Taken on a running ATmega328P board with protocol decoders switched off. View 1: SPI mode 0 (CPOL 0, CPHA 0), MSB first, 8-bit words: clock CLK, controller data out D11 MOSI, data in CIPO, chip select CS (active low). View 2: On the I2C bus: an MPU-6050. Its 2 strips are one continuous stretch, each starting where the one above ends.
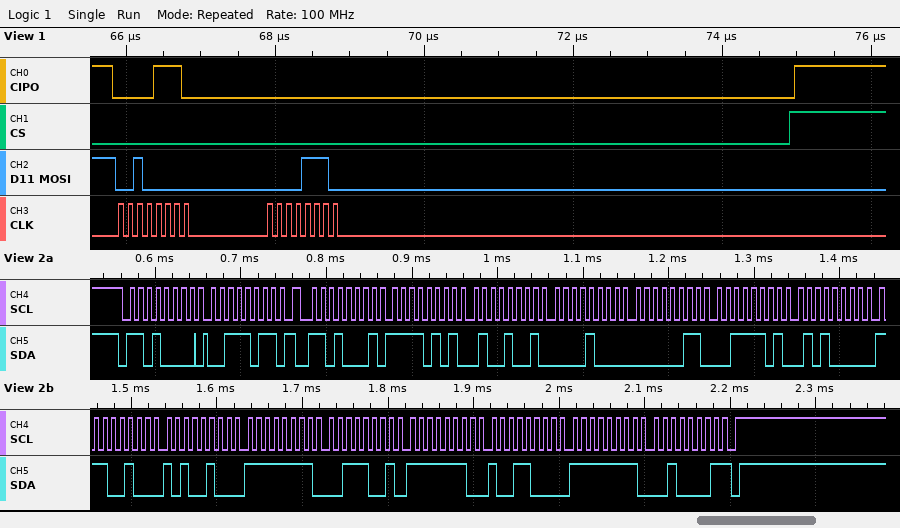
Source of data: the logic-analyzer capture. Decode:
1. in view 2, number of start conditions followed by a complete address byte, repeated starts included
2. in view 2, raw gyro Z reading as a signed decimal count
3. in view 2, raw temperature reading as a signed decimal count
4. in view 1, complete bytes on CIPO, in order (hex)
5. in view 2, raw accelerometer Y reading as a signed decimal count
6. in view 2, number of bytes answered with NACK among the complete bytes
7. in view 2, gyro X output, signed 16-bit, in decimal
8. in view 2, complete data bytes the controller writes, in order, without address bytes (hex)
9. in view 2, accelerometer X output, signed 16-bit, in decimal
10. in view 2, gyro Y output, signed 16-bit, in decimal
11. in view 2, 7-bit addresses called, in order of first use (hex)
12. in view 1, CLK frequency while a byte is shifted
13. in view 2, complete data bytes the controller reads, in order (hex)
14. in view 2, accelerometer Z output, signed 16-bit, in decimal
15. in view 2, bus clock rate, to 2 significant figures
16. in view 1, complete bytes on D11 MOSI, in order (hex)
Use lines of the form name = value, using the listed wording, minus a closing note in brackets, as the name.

in view 2, number of start conditions followed by a complete address byte, repeated starts included = 2
in view 2, raw gyro Z reading as a signed decimal count = -223
in view 2, raw temperature reading as a signed decimal count = -7004
in view 1, complete bytes on CIPO, in order = 0E 00
in view 2, raw accelerometer Y reading as a signed decimal count = 2051
in view 2, number of bytes answered with NACK among the complete bytes = 1
in view 2, gyro X output, signed 16-bit, in decimal = -199
in view 2, complete data bytes the controller writes, in order, without address bytes = 3B
in view 2, accelerometer X output, signed 16-bit, in decimal = -2743
in view 2, gyro Y output, signed 16-bit, in decimal = -360
in view 2, 7-bit addresses called, in order of first use = 0x68
in view 1, CLK frequency while a byte is shifted = 8 MHz
in view 2, complete data bytes the controller reads, in order = F5 49 08 03 3D 50 E4 A4 FF 39 FE 98 FF 21
in view 2, accelerometer Z output, signed 16-bit, in decimal = 15696
in view 2, bus clock rate, to 2 significant figures = 100 kHz
in view 1, complete bytes on D11 MOSI, in order = 20 0E
